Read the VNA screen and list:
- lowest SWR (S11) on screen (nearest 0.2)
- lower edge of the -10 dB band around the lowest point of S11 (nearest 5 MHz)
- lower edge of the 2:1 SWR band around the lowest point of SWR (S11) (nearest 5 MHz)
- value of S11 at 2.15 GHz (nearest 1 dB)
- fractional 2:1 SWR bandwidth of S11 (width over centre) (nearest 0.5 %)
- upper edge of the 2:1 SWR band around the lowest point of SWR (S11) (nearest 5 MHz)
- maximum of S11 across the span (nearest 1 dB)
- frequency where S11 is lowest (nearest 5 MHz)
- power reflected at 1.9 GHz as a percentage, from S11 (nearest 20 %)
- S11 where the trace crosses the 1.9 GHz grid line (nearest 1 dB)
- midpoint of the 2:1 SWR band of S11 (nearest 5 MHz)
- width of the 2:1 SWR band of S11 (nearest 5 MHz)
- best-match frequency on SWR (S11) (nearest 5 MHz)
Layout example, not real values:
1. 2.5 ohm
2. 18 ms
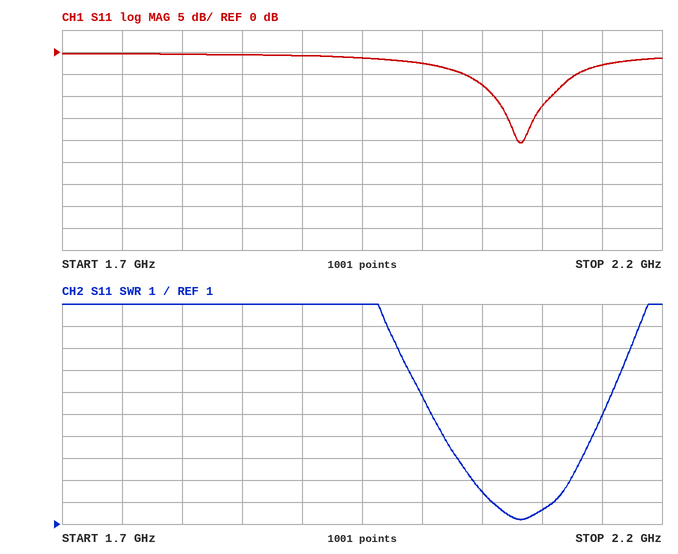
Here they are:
1. 1.2
2. 2.060 GHz
3. 2.060 GHz
4. -3 dB
5. 2.5 %
6. 2.110 GHz
7. 0 dB
8. 2.080 GHz
9. 80 %
10. -1 dB
11. 2.085 GHz
12. 50 MHz
13. 2.080 GHz
